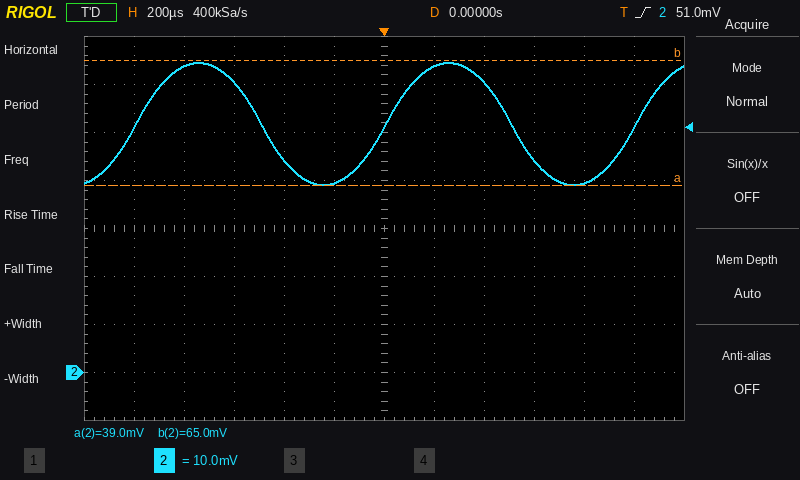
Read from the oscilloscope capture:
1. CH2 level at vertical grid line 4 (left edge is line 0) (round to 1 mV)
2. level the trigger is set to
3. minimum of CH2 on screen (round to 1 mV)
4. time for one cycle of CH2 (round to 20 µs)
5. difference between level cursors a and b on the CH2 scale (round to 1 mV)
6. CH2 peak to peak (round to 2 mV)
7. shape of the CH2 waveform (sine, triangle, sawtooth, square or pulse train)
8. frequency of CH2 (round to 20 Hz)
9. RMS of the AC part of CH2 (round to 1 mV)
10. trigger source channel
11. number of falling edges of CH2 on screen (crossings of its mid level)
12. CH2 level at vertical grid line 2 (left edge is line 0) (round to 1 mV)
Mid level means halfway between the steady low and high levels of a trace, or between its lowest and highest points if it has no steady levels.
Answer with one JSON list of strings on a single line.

["44 mV", "51.0 mV", "39 mV", "1.00 ms", "26 mV", "26 mV", "sine", "1.00 kHz", "9 mV", "CH2", "2", "64 mV"]
